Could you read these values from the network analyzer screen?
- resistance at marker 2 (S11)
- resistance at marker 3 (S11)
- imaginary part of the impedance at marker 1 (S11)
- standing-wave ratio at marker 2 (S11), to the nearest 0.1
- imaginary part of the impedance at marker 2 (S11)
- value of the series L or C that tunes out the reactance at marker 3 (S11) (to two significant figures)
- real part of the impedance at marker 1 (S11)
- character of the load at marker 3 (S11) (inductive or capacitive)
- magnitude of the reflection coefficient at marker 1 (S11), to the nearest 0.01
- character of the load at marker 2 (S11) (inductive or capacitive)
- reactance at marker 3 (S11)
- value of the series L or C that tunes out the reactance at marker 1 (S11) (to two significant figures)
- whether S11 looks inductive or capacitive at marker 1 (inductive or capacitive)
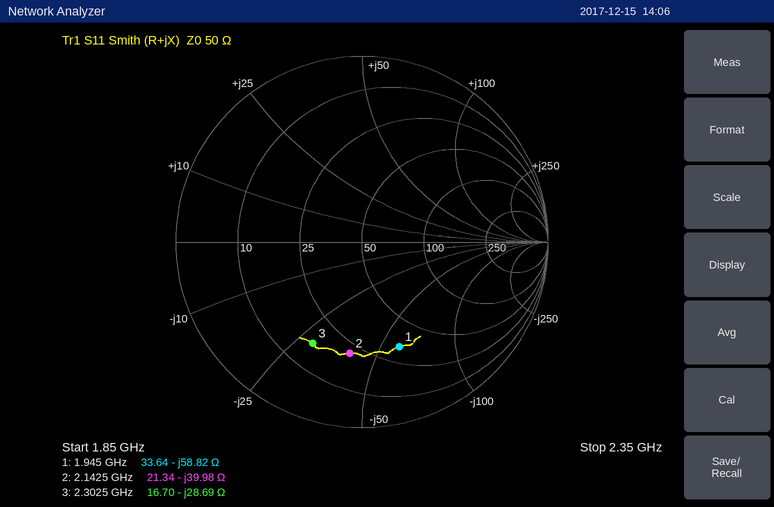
21.34 Ω
16.70 Ω
-58.82 Ω
4.0
-39.98 Ω
2.0 nH
33.64 Ω
capacitive
0.60
capacitive
-28.69 Ω
4.8 nH
capacitive
